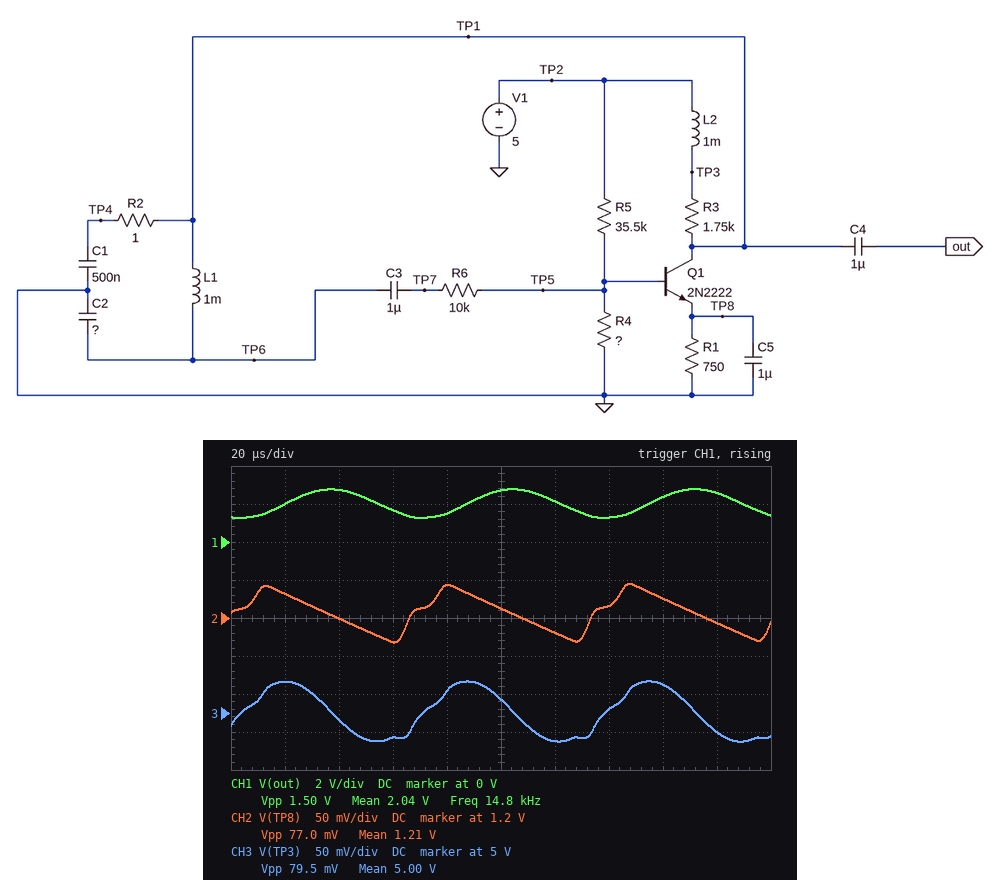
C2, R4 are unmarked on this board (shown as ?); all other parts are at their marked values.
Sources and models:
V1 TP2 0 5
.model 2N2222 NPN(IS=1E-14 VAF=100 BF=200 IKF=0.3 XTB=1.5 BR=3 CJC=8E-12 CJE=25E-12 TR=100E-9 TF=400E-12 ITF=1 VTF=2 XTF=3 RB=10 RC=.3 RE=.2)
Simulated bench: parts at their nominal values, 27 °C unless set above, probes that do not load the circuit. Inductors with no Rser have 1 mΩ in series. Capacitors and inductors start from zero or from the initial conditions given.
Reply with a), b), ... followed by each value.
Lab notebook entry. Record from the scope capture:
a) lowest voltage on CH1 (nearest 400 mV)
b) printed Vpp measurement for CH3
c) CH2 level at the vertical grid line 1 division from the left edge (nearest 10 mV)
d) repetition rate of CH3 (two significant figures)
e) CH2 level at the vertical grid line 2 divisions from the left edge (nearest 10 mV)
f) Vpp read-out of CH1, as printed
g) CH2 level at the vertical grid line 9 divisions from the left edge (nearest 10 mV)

a) 1.2 V
b) 79.5 mV
c) 1.23 V
d) 15 kHz
e) 1.20 V
f) 1.50 V
g) 1.19 V
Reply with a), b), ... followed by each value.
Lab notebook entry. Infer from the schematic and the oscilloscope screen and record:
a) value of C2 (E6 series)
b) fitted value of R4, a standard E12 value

a) 150 nF
b) 8.2 kΩ
